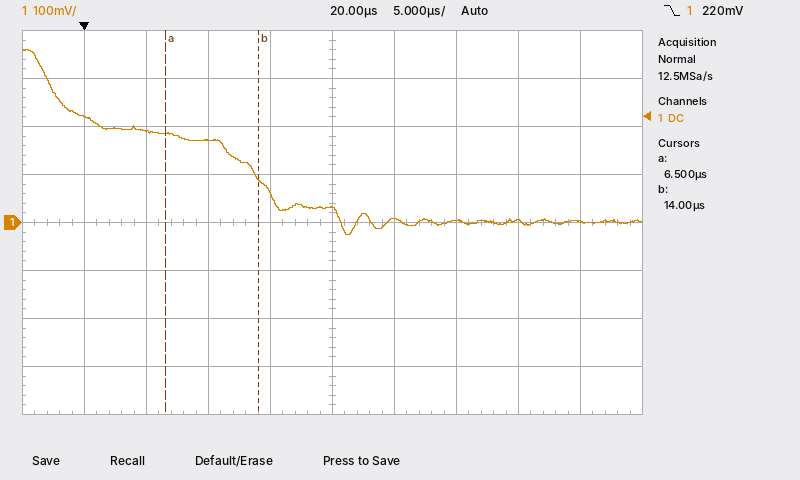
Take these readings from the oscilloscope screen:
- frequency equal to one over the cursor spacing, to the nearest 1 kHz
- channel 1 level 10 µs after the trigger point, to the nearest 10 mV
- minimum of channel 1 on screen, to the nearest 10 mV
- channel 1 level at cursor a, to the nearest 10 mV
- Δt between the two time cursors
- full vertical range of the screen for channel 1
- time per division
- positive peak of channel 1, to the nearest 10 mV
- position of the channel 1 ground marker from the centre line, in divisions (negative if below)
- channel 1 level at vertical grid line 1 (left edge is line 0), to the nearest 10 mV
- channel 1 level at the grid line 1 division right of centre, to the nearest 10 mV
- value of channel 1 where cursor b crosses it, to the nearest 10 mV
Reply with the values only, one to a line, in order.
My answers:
133 kHz
170 mV
-20 mV
190 mV
7.5 µs
800 mV
5 µs
360 mV
0.0 div
220 mV
10 mV
90 mV
